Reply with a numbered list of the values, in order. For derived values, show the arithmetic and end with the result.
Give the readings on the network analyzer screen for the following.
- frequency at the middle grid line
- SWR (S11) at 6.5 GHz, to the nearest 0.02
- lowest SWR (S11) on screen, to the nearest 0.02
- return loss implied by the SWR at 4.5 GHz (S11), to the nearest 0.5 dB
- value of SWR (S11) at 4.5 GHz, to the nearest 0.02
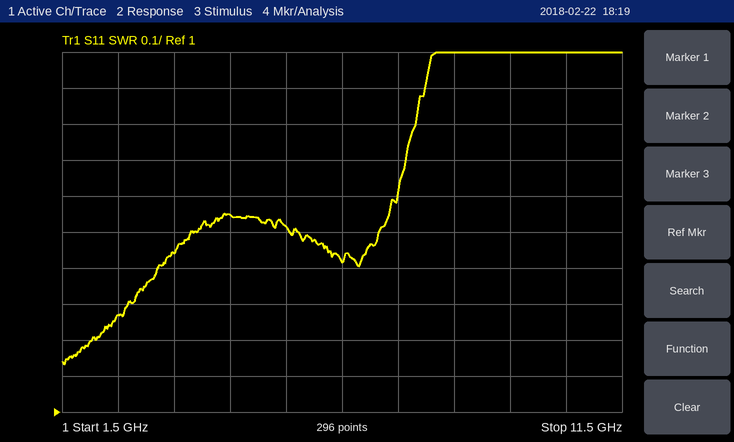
1. 6.5 GHz
2. 1.42
3. 1.14
4. −20 log10((1.54 − 1)/(1.54 + 1)) ≈ 13.4 dB, so 13.5 dB to the nearest 0.5 dB
5. 1.54
